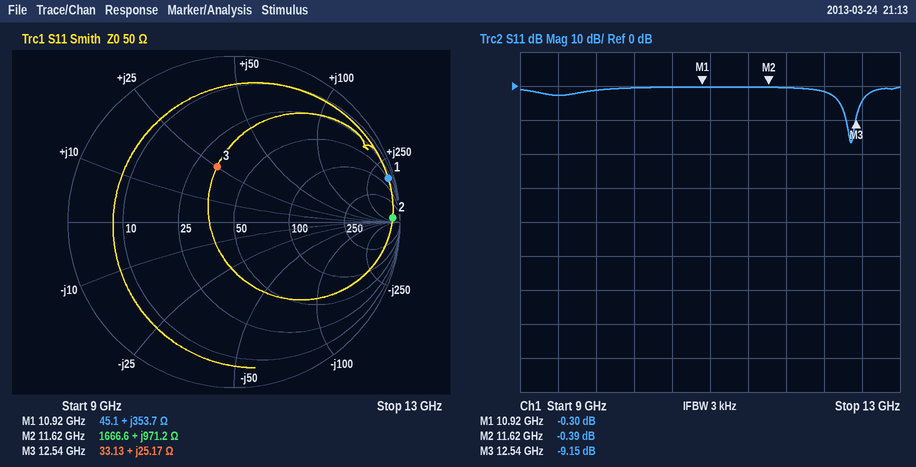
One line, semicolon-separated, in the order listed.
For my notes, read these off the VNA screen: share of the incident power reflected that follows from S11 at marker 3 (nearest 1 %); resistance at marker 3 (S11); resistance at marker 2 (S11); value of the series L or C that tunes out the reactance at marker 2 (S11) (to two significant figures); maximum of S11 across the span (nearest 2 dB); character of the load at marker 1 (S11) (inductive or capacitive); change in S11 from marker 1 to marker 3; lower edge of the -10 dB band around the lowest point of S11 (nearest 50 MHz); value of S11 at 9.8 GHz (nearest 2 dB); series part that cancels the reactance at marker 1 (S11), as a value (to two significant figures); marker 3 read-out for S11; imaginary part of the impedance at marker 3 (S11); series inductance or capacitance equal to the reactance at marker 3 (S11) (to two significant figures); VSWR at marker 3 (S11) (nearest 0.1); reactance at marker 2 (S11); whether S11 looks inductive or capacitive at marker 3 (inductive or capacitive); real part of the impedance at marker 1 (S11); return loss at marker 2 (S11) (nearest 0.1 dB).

12 %; 33.13 Ω; 1666.6 Ω; 14 fF; 0 dB; inductive; -8.85 dB; 12.45 GHz; -2 dB; 41 fF; -9.15 dB; +25.17 Ω; 320 pH; 2.1; +971.2 Ω; inductive; 45.1 Ω; 0.4 dB
